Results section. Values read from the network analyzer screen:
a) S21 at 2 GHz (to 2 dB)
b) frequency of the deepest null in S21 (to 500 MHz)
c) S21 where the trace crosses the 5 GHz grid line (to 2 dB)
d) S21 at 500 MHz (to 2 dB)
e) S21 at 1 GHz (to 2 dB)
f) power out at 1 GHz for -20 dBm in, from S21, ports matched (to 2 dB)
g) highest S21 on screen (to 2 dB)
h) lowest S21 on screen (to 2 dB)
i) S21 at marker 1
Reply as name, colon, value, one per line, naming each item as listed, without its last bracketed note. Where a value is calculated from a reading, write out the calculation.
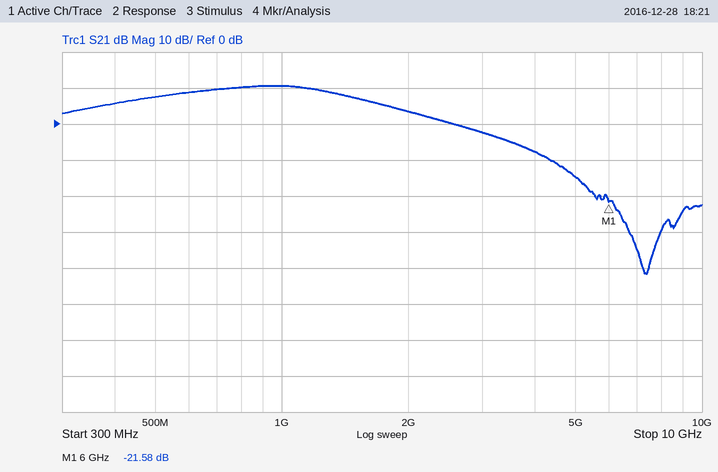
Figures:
S21 at 2 GHz: 4 dB
frequency of the deepest null in S21: 7.5 GHz
S21 where the trace crosses the 5 GHz grid line: -14 dB
S21 at 500 MHz: 8 dB
S21 at 1 GHz: 10 dB
power out at 1 GHz for -20 dBm in, from S21, ports matched: -20 dBm + (10 dB) = -10 dBm
highest S21 on screen: 10 dB
lowest S21 on screen: -42 dB
S21 at marker 1: -21.58 dB
